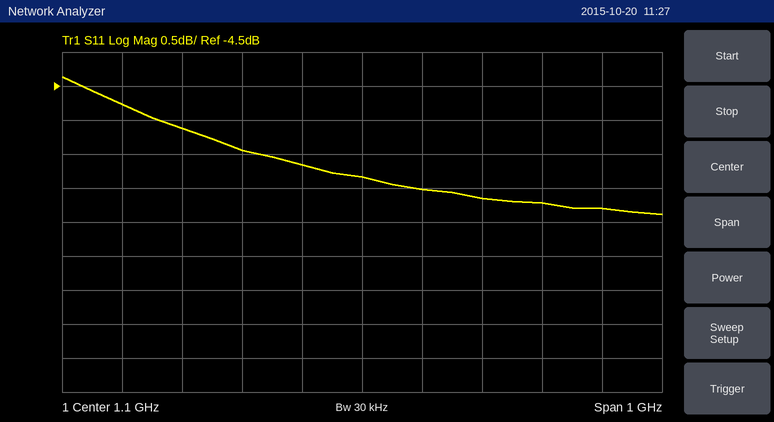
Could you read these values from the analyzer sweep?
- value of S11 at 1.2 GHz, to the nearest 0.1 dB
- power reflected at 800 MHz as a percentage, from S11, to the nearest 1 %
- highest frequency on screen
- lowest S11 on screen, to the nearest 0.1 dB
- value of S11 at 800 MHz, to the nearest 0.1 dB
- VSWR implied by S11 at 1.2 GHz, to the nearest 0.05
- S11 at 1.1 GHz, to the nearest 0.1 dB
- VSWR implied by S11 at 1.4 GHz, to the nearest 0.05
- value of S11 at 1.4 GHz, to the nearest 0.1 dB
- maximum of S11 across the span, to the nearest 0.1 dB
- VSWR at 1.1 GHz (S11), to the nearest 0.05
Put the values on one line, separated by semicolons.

-6.0 dB; 31 %; 1.6 GHz; -6.4 dB; -5.1 dB; 3.00; -5.8 dB; 2.90; -6.2 dB; -4.4 dB; 3.10
